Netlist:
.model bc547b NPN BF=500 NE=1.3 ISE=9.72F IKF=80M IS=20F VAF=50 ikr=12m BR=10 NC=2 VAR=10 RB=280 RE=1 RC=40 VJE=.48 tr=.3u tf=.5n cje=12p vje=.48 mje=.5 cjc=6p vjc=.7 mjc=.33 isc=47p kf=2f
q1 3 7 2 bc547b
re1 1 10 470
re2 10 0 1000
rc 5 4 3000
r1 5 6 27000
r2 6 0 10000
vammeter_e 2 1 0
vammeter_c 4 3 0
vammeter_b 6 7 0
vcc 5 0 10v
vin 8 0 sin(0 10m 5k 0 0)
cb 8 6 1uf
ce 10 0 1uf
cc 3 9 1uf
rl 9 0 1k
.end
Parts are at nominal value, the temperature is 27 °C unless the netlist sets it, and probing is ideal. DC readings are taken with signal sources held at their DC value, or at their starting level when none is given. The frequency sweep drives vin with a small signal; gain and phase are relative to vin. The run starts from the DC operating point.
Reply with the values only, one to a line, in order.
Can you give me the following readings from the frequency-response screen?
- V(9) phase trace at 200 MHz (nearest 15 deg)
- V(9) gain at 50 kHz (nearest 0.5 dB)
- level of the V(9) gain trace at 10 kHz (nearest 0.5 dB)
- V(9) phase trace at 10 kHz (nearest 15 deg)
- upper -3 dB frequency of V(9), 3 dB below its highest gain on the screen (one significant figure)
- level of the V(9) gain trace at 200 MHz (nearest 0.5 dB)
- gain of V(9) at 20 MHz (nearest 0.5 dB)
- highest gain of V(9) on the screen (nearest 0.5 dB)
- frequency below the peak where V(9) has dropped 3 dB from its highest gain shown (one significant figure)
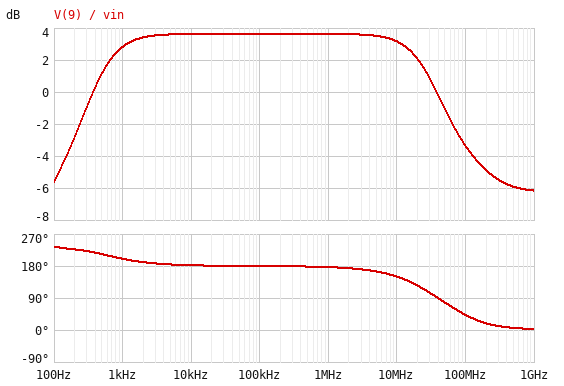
15 deg
3.5 dB
3.5 dB
180 deg
30 MHz
-5.0 dB
2.0 dB
3.5 dB
400 Hz
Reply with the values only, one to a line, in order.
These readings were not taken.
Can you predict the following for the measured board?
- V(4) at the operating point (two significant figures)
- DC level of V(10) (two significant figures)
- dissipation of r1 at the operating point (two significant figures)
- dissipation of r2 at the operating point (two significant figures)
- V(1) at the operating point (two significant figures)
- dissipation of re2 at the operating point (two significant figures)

5.9 V
1.4 V
2.0 mW
710 µW
2.0 V
1.9 mW
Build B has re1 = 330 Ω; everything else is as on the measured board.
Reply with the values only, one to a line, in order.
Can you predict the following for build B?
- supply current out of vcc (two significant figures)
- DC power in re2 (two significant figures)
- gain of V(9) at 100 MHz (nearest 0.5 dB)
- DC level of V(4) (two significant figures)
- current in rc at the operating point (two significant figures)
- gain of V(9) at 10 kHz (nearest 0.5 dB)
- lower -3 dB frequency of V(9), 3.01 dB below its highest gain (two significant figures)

1.8 mA
2.3 mW
-3.0 dB
5.5 V
1.5 mA
6.5 dB
580 Hz
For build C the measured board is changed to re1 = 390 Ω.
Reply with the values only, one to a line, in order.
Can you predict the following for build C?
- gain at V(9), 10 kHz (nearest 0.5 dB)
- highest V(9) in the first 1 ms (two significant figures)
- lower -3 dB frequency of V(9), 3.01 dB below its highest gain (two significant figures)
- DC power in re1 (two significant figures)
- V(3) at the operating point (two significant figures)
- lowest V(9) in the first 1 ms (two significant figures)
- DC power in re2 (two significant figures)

5.0 dB
19 mV
500 Hz
820 µW
5.7 V
-18 mV
2.1 mW
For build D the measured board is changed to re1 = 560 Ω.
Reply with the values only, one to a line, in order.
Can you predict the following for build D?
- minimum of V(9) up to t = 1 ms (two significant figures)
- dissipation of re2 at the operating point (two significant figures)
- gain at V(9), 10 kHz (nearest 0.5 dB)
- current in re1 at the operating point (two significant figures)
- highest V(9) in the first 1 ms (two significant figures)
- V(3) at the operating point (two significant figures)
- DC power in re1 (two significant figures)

-13 mV
1.7 mW
2.0 dB
1.3 mA
13 mV
6.1 V
940 µW
